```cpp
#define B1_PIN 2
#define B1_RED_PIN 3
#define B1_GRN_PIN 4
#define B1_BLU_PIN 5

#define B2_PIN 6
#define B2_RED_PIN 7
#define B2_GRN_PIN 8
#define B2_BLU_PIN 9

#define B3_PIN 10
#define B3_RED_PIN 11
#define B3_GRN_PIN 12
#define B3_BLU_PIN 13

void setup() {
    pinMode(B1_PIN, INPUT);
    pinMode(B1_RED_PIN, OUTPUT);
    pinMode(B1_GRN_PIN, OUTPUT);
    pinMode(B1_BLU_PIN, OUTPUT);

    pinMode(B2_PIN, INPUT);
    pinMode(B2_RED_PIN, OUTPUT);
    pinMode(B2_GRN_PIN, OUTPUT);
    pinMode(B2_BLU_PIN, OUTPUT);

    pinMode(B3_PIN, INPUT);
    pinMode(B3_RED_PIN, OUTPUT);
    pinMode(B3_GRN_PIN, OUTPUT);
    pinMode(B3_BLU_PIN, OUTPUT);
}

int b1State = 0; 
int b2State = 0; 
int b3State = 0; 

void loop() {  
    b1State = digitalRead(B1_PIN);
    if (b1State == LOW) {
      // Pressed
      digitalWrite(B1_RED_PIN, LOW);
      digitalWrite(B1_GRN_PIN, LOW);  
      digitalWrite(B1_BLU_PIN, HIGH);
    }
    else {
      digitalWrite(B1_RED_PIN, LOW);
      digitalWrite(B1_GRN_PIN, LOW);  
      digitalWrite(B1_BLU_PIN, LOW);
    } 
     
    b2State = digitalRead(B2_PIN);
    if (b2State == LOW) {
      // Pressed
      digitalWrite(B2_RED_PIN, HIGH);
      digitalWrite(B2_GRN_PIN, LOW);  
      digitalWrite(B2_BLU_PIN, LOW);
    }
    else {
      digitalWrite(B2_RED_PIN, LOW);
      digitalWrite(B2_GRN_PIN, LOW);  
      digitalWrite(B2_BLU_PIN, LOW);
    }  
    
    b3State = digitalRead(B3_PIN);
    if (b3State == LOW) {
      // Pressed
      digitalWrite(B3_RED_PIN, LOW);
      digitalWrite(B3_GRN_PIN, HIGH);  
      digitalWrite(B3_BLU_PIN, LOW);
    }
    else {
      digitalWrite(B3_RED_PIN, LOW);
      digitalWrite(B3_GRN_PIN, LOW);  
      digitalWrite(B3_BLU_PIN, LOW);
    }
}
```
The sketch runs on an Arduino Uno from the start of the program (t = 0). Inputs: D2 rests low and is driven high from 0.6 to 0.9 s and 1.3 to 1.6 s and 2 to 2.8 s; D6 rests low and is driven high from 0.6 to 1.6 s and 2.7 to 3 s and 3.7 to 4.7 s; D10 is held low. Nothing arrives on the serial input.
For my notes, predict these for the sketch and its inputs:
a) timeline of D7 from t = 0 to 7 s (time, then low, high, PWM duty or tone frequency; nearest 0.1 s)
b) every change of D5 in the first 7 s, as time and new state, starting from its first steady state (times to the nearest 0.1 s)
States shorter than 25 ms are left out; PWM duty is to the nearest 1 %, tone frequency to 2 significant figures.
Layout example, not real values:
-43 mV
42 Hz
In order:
0 s high; 0.6 s low; 1.6 s high; 2.7 s low; 3 s high; 3.7 s low; 4.7 s high
0 s high; 0.6 s low; 0.9 s high; 1.3 s low; 1.6 s high; 2 s low; 2.8 s high
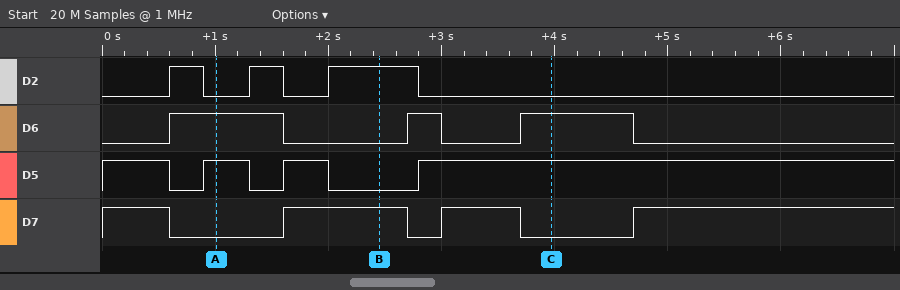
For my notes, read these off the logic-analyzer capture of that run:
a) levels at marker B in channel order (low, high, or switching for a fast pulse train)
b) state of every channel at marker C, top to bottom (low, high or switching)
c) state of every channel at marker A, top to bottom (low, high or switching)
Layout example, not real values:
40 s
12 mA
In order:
D2 high, D6 low, D5 low, D7 high
D2 low, D6 high, D5 high, D7 low
D2 low, D6 high, D5 high, D7 low
